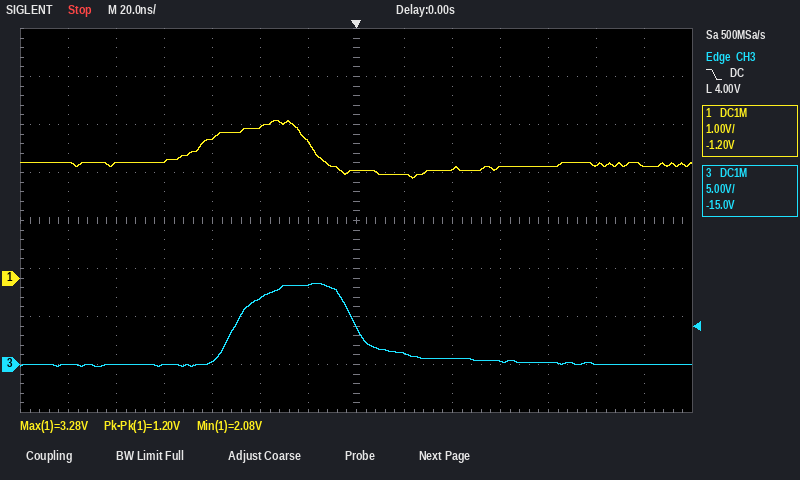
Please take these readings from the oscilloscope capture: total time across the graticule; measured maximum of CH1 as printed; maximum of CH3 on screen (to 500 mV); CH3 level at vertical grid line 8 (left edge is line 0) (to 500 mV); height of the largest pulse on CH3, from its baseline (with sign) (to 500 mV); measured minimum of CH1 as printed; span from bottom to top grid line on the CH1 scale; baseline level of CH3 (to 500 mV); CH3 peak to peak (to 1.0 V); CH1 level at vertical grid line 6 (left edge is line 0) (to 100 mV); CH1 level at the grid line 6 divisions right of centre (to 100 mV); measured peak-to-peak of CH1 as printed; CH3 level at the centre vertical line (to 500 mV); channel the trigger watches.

280 ns
3.28 V
8.5 V
1.0 V
+8.5 V
2.08 V
8 V
0.0 V
9.0 V
2.8 V
2.3 V
1.20 V
4.0 V
CH3
